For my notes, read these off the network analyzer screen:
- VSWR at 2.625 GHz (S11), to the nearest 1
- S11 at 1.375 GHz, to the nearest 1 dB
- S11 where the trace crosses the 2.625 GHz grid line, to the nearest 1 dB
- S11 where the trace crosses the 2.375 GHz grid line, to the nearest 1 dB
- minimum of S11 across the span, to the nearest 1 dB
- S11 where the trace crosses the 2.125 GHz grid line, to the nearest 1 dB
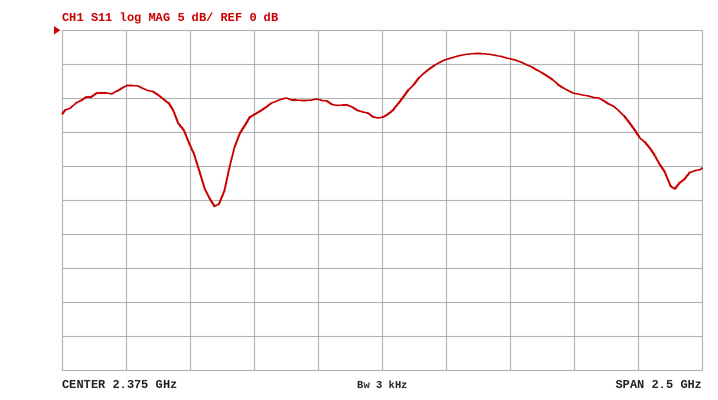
4
-8 dB
-4 dB
-13 dB
-26 dB
-10 dB
